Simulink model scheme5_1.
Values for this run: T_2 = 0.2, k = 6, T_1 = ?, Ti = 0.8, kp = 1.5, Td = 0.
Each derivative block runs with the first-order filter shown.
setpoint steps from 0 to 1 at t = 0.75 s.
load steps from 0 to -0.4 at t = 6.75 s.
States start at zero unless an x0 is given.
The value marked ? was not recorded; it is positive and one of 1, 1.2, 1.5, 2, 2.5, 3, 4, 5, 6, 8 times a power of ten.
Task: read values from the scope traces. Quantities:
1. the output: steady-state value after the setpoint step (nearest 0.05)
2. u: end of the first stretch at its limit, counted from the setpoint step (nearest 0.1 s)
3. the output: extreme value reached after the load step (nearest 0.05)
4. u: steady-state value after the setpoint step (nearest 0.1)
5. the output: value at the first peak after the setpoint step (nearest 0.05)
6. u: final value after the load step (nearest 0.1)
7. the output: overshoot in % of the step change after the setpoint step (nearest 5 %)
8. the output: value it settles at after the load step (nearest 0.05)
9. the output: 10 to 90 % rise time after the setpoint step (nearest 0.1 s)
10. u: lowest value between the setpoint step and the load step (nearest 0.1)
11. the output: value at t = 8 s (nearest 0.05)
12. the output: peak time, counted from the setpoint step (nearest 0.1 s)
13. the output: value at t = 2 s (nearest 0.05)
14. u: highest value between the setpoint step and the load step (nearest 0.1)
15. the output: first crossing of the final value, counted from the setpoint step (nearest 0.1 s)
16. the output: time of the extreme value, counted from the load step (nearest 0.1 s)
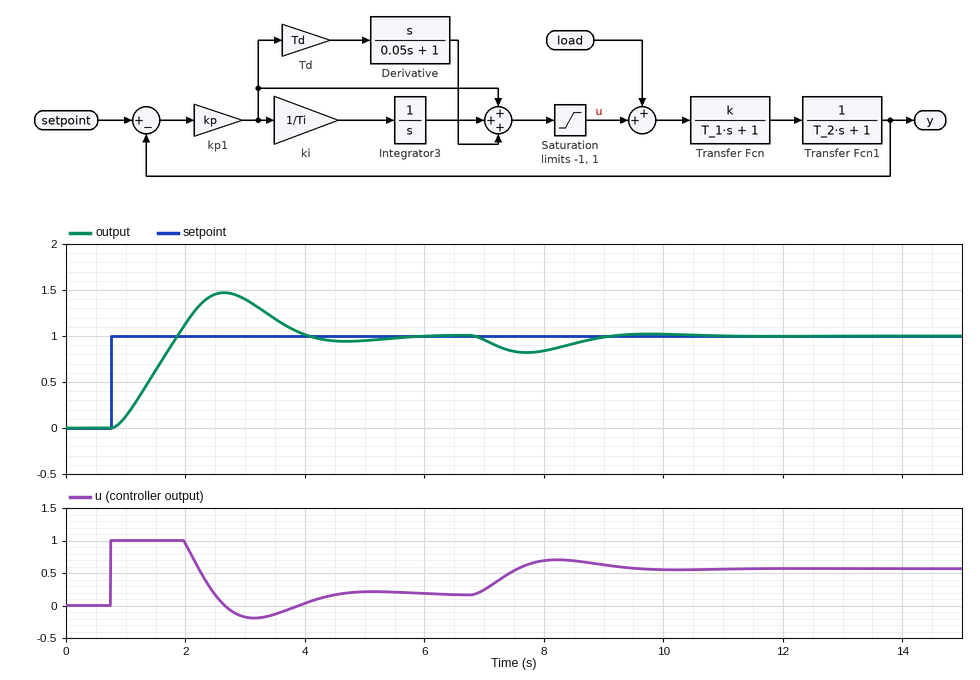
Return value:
1.00
1.2 s
0.80
0.2
1.45
0.6
45 %
1.00
0.8 s
-0.2
0.85
1.9 s
1.15
1.0
1.1 s
1.0 s
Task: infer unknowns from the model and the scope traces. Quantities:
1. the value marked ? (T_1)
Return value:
5
